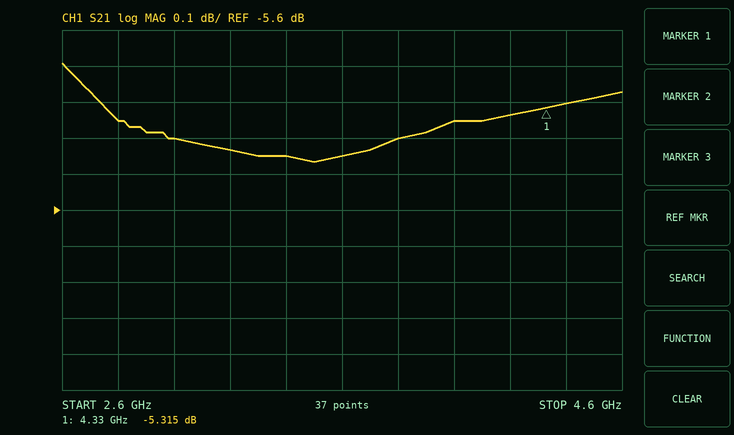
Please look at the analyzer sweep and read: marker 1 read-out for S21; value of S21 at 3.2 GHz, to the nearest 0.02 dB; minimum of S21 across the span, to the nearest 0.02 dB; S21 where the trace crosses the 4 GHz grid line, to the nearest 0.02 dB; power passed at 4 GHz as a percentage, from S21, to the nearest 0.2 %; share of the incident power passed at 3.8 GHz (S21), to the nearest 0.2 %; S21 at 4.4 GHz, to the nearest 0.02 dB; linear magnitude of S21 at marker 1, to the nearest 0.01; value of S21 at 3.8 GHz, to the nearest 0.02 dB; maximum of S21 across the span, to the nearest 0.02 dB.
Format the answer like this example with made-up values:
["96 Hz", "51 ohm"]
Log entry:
["-5.315 dB", "-5.44 dB", "-5.46 dB", "-5.36 dB", "29.2 %", "28.8 %", "-5.30 dB", "0.54", "-5.40 dB", "-5.20 dB"]
